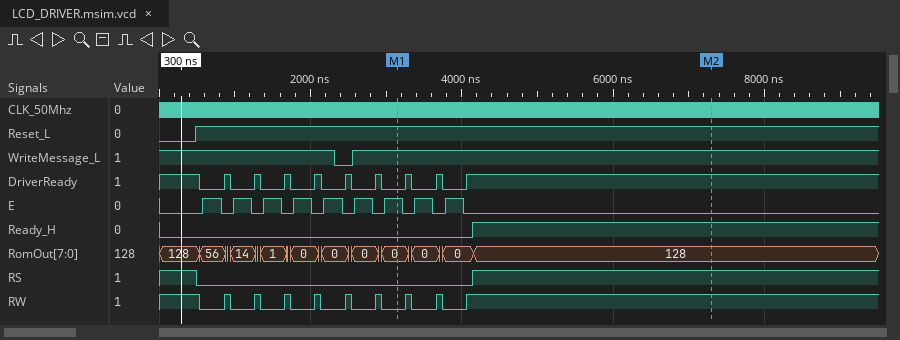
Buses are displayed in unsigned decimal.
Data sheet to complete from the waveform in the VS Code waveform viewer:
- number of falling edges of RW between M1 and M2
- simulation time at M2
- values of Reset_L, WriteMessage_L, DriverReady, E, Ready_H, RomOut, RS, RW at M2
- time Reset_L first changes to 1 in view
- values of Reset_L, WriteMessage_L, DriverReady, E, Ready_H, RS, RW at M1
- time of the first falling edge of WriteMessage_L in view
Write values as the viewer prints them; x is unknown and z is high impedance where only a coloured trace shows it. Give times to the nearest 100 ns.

2
7300 ns
Reset_L=1, WriteMessage_L=1, DriverReady=1, E=0, Ready_H=1, RomOut=128, RS=1, RW=1
500 ns
Reset_L=1, WriteMessage_L=1, DriverReady=0, E=1, Ready_H=0, RS=0, RW=0
2300 ns
